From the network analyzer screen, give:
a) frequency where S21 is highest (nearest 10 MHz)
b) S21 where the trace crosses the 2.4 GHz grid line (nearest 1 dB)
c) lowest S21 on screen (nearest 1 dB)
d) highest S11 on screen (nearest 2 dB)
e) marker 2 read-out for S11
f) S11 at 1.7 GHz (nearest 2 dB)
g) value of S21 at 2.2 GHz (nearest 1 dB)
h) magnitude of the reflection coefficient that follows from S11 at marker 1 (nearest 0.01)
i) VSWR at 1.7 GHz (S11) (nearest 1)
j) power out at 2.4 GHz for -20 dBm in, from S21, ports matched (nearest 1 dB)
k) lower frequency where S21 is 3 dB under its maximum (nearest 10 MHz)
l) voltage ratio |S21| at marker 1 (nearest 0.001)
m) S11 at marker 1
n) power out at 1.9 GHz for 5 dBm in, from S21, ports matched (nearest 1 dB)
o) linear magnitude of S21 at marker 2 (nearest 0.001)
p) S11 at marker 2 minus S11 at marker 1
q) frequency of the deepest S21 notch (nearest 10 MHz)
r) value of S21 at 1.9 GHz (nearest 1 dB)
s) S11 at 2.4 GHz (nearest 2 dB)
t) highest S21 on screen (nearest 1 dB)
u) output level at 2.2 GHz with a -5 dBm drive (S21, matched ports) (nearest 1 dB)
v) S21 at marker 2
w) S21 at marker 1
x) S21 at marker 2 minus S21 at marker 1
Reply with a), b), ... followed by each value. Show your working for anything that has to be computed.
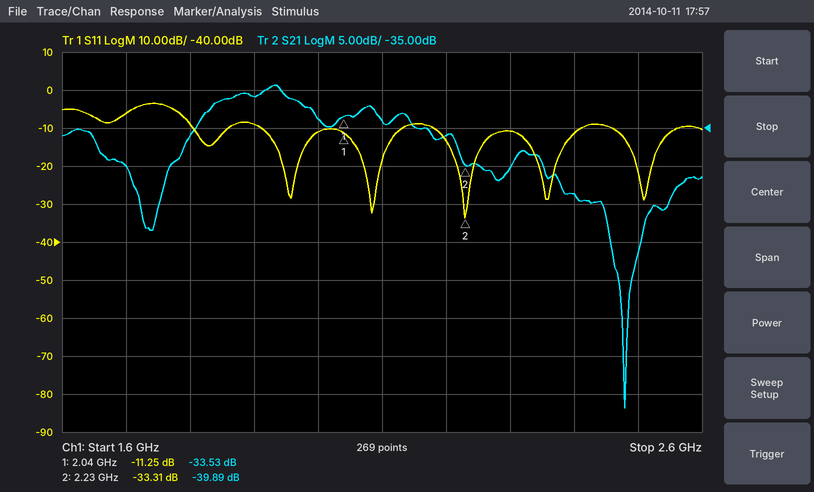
a) 1.93 GHz
b) -44 dB
c) -72 dB
d) -4 dB
e) -33.31 dB
f) -6 dB
g) -36 dB
h) 10^(-11.25/20) ≈ 0.27
i) |Γ| = 10^(-6/20) = 0.5012; VSWR = (1 + 0.5012)/(1 − 0.5012) ≈ 3
j) -20 dBm + (-44 dB) = -64 dBm
k) 1.83 GHz
l) 10^(-33.53/20) ≈ 0.021
m) -11.25 dB
n) 5 dBm + (-31 dB) = -26 dBm
o) 10^(-39.89/20) ≈ 0.010
p) -33.31 − (-11.25) = -22.06 dB
q) 2.48 GHz
r) -31 dB
s) -12 dB
t) -29 dB
u) -5 dBm + (-36 dB) = -41 dBm
v) -39.89 dB
w) -33.53 dB
x) -39.89 − (-33.53) = -6.36 dB
